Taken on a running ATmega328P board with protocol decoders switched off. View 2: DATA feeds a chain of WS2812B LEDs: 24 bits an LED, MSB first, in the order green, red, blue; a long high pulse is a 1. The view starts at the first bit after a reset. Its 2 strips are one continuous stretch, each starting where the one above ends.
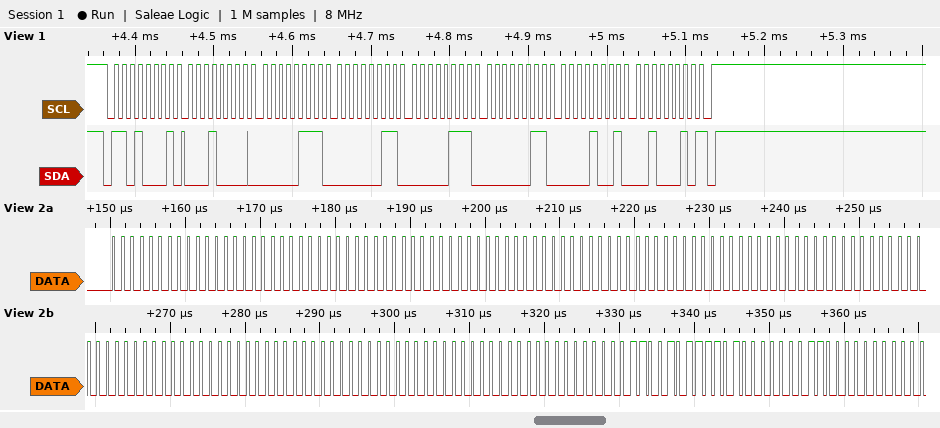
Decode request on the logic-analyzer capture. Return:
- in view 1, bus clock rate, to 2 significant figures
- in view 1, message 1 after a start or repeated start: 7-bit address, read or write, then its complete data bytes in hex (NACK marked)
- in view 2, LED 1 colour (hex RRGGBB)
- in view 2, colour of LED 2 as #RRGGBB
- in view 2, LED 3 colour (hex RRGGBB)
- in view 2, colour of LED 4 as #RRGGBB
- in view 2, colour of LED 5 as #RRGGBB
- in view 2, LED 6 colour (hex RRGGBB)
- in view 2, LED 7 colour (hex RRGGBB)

100 kHz
0x68 read: 10 07 03 07 03 09 22 NACK
#000000
#000000
#000000
#000000
#000000
#000000
#E8650C
